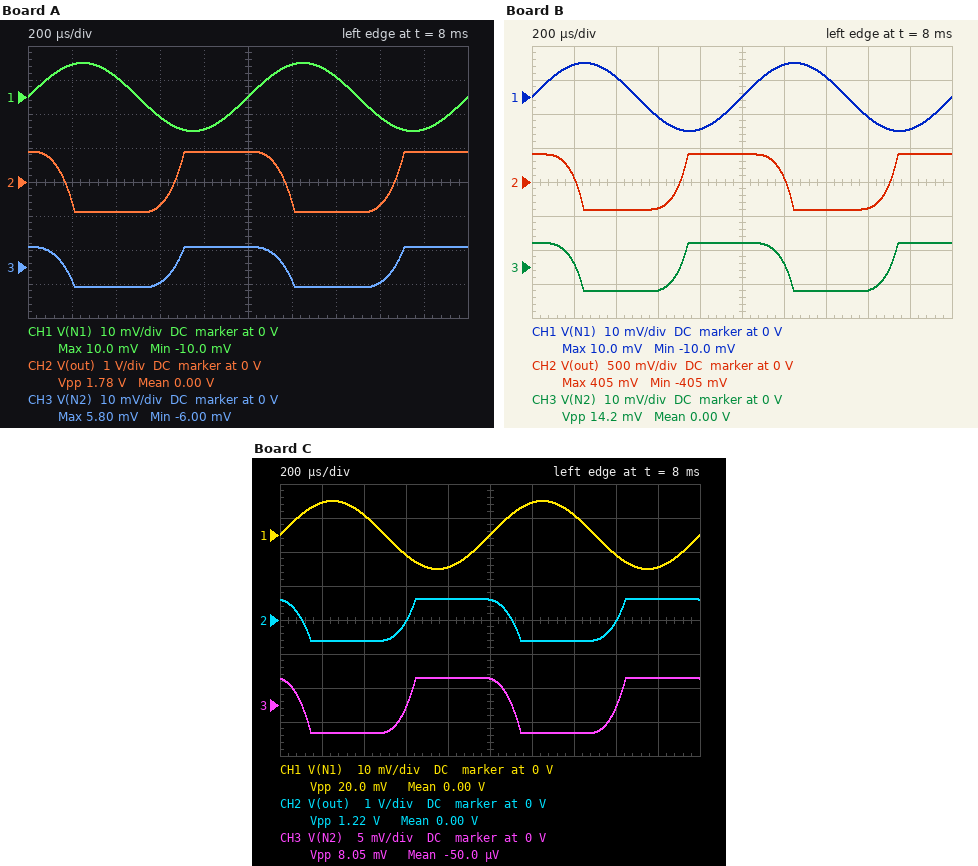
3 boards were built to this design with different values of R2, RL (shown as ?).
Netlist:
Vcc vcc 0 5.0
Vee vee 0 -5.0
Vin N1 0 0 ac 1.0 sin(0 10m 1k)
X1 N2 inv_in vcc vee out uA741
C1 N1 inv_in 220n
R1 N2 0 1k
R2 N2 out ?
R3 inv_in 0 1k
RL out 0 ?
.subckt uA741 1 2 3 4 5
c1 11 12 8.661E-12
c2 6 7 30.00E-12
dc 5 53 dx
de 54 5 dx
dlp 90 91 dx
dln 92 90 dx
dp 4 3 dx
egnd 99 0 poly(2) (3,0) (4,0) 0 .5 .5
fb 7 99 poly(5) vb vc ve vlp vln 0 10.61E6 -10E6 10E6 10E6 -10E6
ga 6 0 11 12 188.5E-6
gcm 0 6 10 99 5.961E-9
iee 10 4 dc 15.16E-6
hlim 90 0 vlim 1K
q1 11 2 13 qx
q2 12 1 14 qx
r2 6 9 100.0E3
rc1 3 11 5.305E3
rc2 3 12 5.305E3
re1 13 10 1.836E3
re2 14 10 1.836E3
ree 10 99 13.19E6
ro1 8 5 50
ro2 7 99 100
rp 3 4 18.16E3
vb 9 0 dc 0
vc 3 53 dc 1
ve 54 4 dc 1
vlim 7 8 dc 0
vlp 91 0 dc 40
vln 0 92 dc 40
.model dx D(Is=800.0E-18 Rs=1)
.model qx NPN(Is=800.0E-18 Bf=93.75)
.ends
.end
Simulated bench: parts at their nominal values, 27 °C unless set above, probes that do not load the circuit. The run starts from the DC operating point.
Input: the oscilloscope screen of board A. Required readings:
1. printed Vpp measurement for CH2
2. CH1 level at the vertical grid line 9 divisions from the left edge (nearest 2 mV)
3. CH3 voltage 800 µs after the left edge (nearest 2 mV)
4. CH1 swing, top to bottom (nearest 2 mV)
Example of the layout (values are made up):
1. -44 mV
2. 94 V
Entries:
1. 1.78 V
2. -10 mV
3. 6 mV
4. 20 mV
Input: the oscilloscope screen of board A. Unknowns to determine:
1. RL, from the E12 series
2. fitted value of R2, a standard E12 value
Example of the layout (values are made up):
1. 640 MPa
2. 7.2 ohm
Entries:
1. 22 Ω
2. 150 kΩ
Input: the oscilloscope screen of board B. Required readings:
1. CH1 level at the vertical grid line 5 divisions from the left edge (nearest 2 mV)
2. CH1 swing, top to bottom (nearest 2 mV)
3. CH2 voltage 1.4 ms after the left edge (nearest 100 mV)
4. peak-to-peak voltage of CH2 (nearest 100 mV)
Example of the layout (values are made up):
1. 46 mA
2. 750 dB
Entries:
1. 0 V
2. 20 mV
3. -400 mV
4. 800 mV
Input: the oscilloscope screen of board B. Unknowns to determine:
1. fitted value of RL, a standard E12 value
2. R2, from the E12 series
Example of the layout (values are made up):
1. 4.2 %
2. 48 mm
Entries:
1. 10 Ω
2. 56 kΩ
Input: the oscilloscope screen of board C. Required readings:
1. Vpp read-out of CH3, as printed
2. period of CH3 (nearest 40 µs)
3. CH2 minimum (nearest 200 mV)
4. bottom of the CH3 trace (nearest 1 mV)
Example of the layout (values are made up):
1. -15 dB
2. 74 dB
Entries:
1. 8.05 mV
2. 1.00 ms
3. -600 mV
4. -4 mV
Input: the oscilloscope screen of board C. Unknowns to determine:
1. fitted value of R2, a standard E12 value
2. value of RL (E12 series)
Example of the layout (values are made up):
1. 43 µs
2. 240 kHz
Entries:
1. 150 kΩ
2. 15 Ω
